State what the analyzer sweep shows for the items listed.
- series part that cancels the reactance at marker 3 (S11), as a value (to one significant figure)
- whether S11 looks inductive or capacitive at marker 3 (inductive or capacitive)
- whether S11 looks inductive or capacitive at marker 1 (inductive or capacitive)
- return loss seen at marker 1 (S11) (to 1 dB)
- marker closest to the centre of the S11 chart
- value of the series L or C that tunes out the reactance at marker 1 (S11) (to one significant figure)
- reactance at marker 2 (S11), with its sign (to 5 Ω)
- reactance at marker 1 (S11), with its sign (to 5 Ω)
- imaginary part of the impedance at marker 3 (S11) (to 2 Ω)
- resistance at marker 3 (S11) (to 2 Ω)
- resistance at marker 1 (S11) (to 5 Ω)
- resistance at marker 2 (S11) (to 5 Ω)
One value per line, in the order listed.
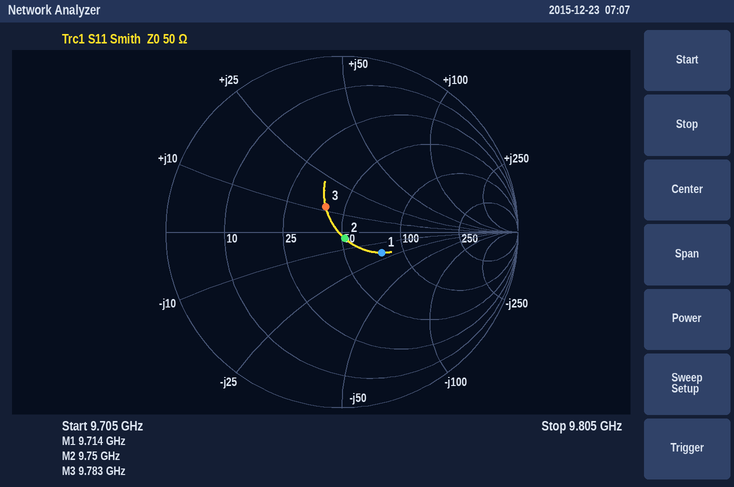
1 pF
inductive
capacitive
12 dB
marker 2
300 pH
-5 Ω
-20 Ω
+12 Ω
40 Ω
75 Ω
50 Ω
